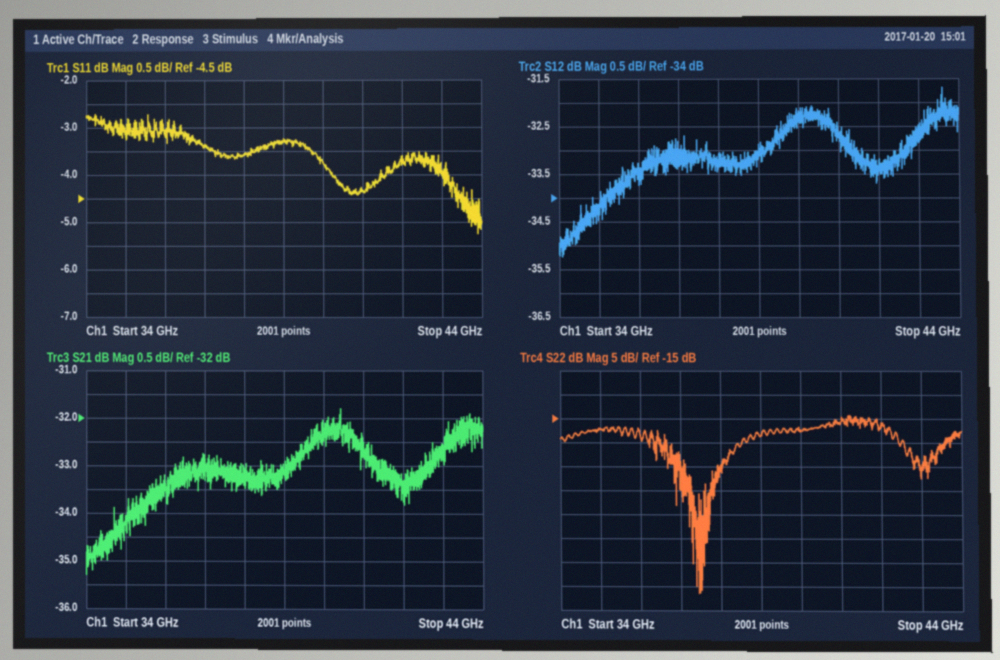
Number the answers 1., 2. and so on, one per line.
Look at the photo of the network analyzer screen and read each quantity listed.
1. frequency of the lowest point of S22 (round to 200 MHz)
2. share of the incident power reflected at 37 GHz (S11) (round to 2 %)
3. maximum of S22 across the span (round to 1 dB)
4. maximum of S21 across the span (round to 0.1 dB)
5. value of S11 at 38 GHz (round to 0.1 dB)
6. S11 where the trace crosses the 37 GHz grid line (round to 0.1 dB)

1. 37.4 GHz
2. 46 %
3. -14 dB
4. -31.8 dB
5. -3.6 dB
6. -3.4 dB
